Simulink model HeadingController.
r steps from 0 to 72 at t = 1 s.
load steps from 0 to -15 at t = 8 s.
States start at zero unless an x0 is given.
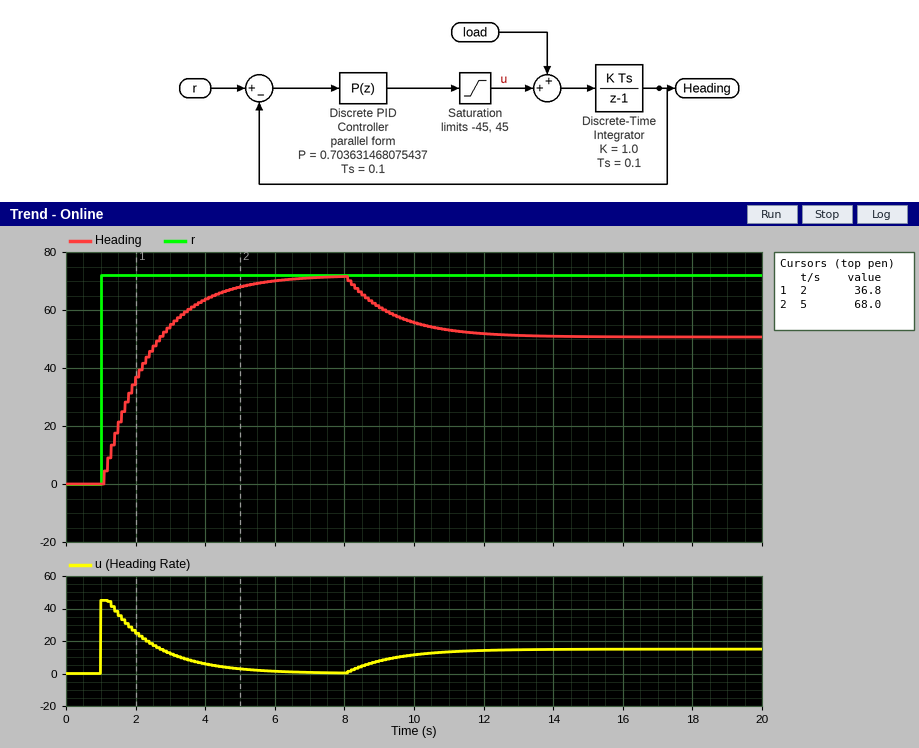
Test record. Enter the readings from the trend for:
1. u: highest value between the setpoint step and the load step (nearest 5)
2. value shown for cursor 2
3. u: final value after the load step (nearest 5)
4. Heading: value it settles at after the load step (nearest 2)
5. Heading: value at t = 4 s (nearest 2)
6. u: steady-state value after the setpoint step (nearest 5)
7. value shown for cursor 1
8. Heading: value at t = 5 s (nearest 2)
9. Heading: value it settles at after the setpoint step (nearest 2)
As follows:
45
68.0
15
50
64
0
36.8
68
72
